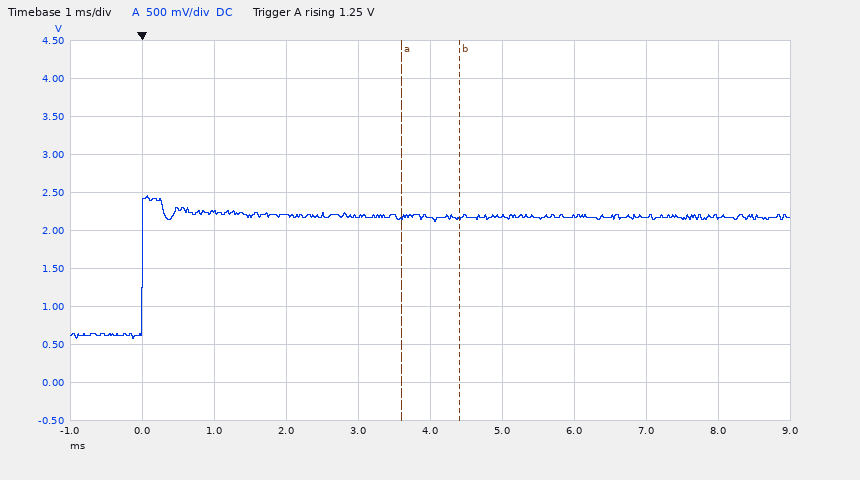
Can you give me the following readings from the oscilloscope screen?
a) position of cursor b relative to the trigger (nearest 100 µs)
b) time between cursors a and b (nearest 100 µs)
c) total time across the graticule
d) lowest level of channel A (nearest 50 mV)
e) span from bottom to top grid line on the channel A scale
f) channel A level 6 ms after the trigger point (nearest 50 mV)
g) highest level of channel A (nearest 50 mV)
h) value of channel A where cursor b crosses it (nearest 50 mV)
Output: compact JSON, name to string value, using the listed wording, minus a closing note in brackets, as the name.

{"position of cursor b relative to the trigger": "+4.4 ms", "time between cursors a and b": "800 µs", "total time across the graticule": "10 ms", "lowest level of channel A": "600 mV", "span from bottom to top grid line on the channel A scale": "5 V", "channel A level 6 ms after the trigger point": "2.20 V", "highest level of channel A": "2.45 V", "value of channel A where cursor b crosses it": "2.15 V"}
